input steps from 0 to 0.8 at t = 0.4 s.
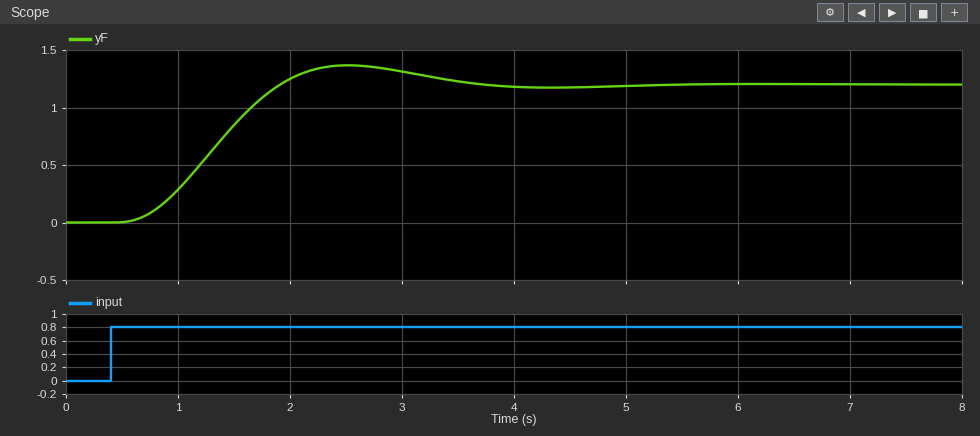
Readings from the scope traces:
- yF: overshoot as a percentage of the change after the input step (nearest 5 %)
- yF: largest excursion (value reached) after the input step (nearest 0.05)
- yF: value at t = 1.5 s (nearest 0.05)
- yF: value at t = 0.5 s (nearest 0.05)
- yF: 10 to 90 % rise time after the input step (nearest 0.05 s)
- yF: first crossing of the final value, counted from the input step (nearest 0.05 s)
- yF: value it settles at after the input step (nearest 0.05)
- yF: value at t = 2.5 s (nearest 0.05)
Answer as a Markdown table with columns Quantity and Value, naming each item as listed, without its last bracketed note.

| Quantity | Value |
|---|---|
| yF: overshoot as a percentage of the change after the input step | 15 % |
| yF: largest excursion (value reached) after the input step | 1.35 |
| yF: value at t = 1.5 s | 0.85 |
| yF: value at t = 0.5 s | 0.00 |
| yF: 10 to 90 % rise time after the input step | 0.95 s |
| yF: first crossing of the final value, counted from the input step | 1.50 s |
| yF: value it settles at after the input step | 1.20 |
| yF: value at t = 2.5 s | 1.35 |
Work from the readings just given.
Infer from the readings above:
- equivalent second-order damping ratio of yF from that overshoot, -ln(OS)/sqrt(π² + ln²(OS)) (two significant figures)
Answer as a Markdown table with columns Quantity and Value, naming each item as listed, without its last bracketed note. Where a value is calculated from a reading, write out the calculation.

| Quantity | Value |
|---|---|
| equivalent second-order damping ratio of yF from that overshoot, -ln(OS)/sqrt(π² + ln²(OS)) | ln(0.15) = -1.897; 1.897 / sqrt(9.870 + 3.599) = 0.52 |
